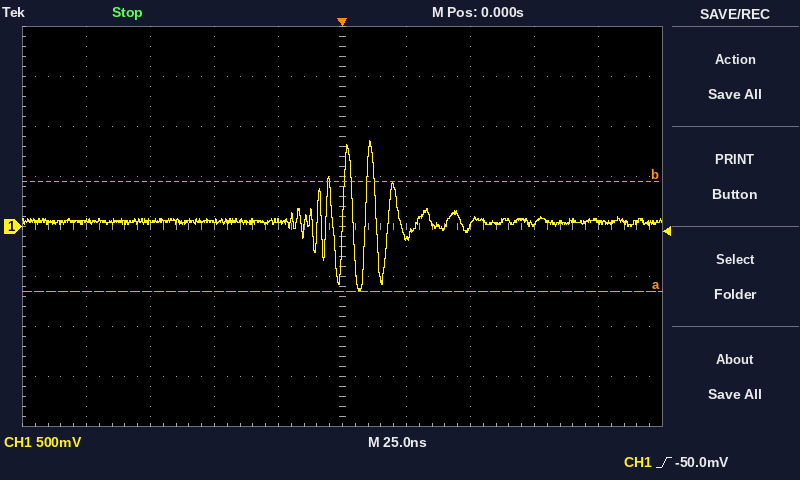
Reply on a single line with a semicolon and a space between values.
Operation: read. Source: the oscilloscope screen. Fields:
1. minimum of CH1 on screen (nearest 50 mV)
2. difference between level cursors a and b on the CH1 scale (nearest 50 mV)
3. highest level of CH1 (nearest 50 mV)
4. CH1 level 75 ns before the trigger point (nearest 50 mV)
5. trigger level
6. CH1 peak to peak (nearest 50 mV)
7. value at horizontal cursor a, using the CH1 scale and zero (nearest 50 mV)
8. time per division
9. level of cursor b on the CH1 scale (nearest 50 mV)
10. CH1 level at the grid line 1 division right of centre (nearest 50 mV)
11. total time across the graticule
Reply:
-650 mV; 1.10 V; 850 mV; 50 mV; -50.0 mV; 1.50 V; -650 mV; 25 ns; 450 mV; -100 mV; 250 ns
